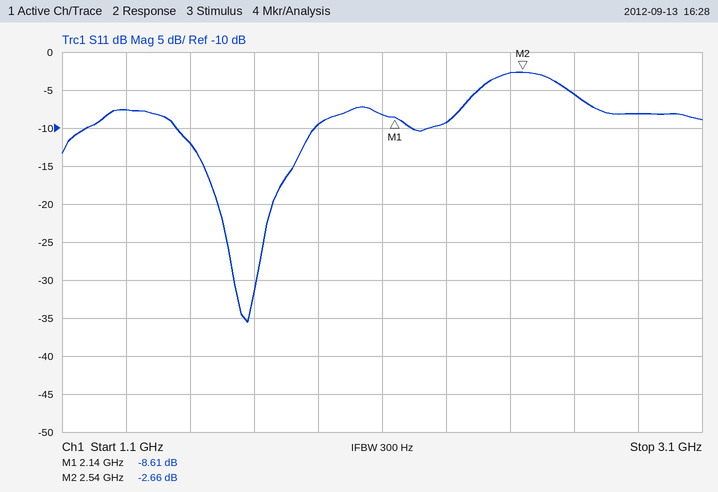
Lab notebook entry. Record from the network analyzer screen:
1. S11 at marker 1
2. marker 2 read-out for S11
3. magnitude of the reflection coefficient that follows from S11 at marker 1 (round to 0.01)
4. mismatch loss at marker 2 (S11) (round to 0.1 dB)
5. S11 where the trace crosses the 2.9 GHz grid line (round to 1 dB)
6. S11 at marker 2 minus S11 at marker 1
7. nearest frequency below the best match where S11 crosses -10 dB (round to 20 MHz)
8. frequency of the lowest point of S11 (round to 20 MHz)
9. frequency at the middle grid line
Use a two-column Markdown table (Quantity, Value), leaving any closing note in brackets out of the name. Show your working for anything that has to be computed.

| Quantity | Value |
|---|---|
| S11 at marker 1 | -8.61 dB |
| marker 2 read-out for S11 | -2.66 dB |
| magnitude of the reflection coefficient that follows from S11 at marker 1 | 10^(-8.61/20) ≈ 0.37 |
| mismatch loss at marker 2 (S11) | −10 log10(1 − 10^(-2.66/10)) ≈ 3.4 dB |
| S11 where the trace crosses the 2.9 GHz grid line | -8 dB |
| S11 at marker 2 minus S11 at marker 1 | -2.66 − (-8.61) = 5.95 dB |
| nearest frequency below the best match where S11 crosses -10 dB | 1.46 GHz |
| frequency of the lowest point of S11 | 1.68 GHz |
| frequency at the middle grid line | 2.1 GHz |
